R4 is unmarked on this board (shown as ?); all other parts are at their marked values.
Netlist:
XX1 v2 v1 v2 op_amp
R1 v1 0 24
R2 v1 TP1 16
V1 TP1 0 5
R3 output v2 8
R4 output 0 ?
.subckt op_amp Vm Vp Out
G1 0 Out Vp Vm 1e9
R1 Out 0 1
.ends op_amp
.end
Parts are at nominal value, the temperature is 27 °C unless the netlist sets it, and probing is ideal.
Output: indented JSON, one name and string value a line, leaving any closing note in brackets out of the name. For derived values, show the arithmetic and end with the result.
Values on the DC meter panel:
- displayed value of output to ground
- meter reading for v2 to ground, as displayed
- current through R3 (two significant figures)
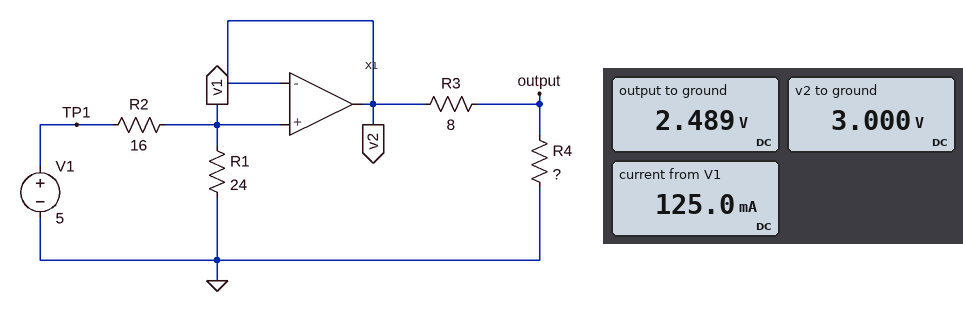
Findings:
{
  "displayed value of output to ground": "2.489 V",
  "meter reading for v2 to ground, as displayed": "3.000 V",
  "current through R3": "(3 V - 2.489 V) / 8 Ω = 64 mA"
}
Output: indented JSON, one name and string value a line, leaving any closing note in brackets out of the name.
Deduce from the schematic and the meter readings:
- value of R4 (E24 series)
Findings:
{
  "value of R4": "39 Ω"
}
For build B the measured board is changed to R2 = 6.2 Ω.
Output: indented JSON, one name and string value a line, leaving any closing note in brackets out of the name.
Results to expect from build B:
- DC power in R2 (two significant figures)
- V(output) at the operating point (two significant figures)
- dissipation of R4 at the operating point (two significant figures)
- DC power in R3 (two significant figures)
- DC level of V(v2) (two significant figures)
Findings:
{
  "DC power in R2": "170 mW",
  "V(output) at the operating point": "3.3 V",
  "dissipation of R4 at the operating point": "280 mW",
  "DC power in R3": "57 mW",
  "DC level of V(v2)": "4.0 V"
}
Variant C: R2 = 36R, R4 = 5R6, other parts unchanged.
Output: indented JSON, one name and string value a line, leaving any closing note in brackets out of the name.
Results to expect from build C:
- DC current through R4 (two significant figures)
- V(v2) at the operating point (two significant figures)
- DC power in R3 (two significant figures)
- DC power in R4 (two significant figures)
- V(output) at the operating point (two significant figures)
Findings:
{
  "DC current through R4": "150 mA",
  "V(v2) at the operating point": "2.0 V",
  "DC power in R3": "170 mW",
  "DC power in R4": "120 mW",
  "V(output) at the operating point": "820 mV"
}
